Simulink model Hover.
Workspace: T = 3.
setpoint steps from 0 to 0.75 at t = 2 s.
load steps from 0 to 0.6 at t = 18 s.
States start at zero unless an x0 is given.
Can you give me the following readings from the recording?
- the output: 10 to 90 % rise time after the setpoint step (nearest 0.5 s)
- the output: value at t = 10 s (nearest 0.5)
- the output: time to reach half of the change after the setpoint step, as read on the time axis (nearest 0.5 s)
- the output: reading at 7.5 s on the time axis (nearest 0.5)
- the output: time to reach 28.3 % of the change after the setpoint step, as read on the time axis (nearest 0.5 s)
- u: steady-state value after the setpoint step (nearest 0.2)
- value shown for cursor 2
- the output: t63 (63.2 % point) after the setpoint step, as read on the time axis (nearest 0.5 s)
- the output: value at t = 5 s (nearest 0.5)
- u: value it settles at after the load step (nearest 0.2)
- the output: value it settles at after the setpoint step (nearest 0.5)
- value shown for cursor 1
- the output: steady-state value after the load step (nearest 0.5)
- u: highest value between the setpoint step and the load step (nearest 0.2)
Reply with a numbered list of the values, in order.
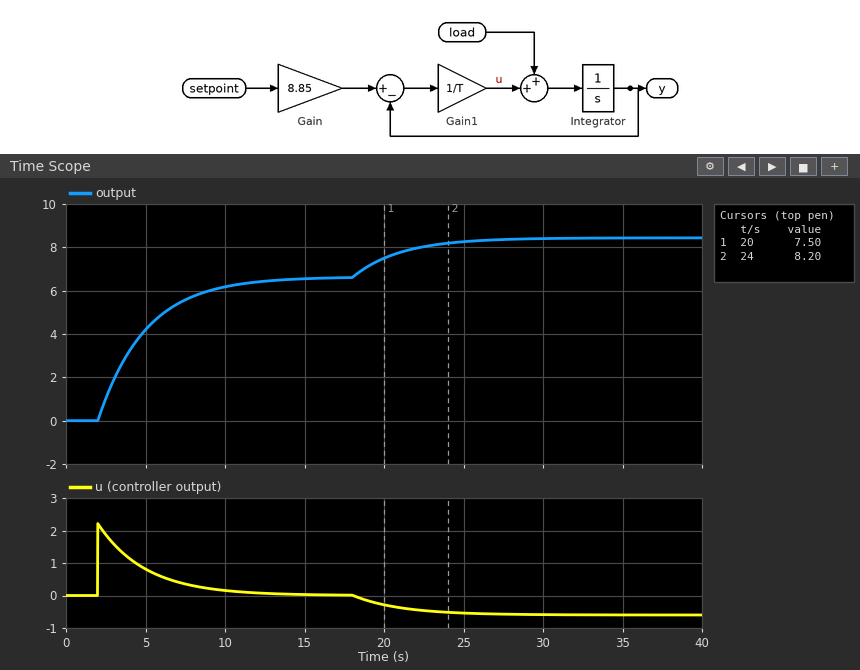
1. 6.5 s
2. 6.0
3. 4.0 s
4. 5.5
5. 3.0 s
6. 0.0
7. 8.20
8. 5.0 s
9. 4.0
10. -0.6
11. 6.5
12. 7.50
13. 8.5
14. 2.2
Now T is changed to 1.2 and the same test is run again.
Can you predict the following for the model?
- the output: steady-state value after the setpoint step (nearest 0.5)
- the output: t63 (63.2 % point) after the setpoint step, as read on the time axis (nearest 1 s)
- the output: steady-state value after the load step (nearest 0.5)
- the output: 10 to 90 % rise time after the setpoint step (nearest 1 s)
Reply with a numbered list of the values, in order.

1. 6.5
2. 3 s
3. 7.5
4. 3 s
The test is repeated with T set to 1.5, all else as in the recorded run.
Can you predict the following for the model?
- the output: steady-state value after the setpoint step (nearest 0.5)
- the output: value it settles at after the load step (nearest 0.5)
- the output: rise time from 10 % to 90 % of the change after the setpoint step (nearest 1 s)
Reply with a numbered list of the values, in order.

1. 6.5
2. 7.5
3. 3 s
